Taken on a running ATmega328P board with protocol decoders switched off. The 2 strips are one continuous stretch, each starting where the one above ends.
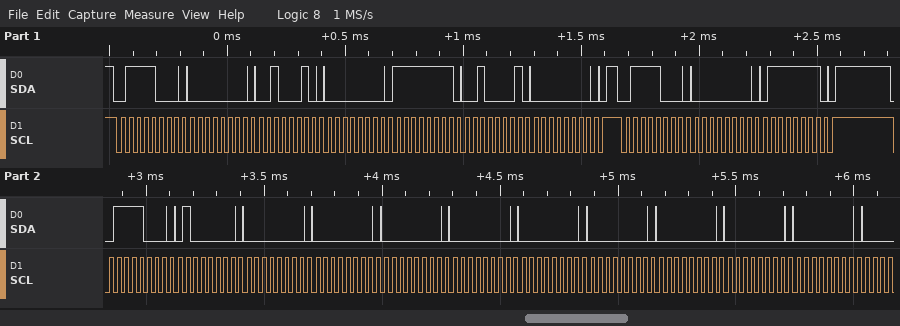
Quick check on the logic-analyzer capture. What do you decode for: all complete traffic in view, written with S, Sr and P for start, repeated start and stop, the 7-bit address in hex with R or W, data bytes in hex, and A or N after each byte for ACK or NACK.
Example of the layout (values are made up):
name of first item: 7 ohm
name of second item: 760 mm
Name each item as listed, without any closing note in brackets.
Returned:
all complete traffic in view, written with S, Sr and P for start, repeated start and stop, the 7-bit address in hex with R or W, data bytes in hex, and A or N after each byte for ACK or NACK: S 3CW A 00 A 22 A 00 A FF A 21 A 00 A P S 3CW A 00 A 7F A P S 3CW A 40 A 00 A 00 A 00 A 00 A 00 A 00 A 00 A 00 A 00 A
